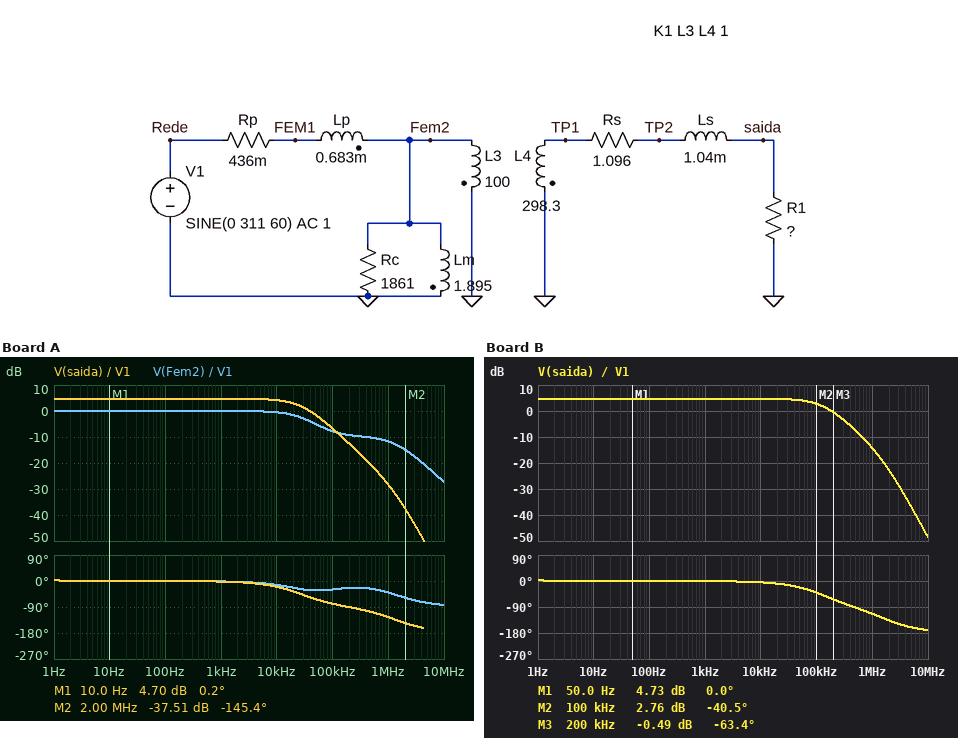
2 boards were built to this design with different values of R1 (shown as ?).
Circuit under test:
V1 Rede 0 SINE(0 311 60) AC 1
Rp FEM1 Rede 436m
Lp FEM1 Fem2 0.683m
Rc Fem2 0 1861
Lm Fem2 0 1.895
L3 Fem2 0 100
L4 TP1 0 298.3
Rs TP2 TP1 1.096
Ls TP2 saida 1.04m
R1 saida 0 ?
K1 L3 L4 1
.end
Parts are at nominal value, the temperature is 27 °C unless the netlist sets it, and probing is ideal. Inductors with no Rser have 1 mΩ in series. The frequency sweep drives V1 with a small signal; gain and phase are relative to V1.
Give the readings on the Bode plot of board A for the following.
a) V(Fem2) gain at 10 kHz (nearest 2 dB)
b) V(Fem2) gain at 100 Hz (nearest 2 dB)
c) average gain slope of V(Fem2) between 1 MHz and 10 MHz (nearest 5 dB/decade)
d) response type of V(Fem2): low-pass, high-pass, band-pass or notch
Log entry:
0 dB
0 dB
-15 dB/decade
low-pass
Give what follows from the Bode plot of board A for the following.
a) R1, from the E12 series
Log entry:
560 Ω
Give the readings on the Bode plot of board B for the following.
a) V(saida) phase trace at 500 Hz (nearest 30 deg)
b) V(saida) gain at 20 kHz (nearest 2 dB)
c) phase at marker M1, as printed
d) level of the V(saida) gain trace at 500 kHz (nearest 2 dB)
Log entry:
0 deg
4 dB
0.0 deg
-8 dB
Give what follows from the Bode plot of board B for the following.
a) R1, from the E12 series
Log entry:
3.3 kΩ
